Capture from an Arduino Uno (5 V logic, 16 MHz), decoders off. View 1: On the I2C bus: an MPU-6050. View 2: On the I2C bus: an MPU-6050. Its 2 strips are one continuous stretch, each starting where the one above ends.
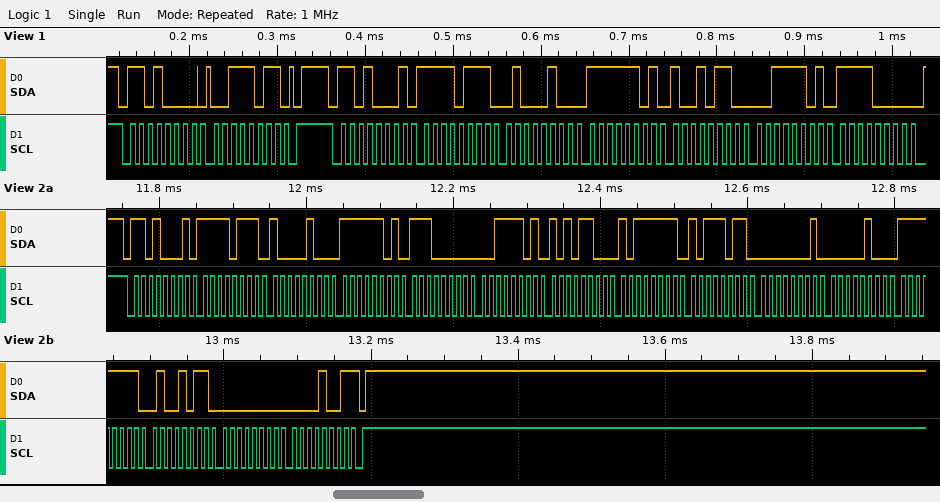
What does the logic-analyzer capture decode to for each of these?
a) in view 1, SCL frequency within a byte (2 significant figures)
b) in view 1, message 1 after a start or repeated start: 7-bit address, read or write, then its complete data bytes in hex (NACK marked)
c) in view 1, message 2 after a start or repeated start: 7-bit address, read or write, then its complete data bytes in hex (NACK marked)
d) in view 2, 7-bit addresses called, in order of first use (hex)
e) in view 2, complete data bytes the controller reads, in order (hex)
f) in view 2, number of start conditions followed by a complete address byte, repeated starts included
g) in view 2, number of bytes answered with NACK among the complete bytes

100 kHz
0x68 write: 3B
0x68 read: F7 44 FD 96 3D F0
0x68
F7 84 FD E0 3D AC BF BB 01 04 FF 4B 00 09
1
1
